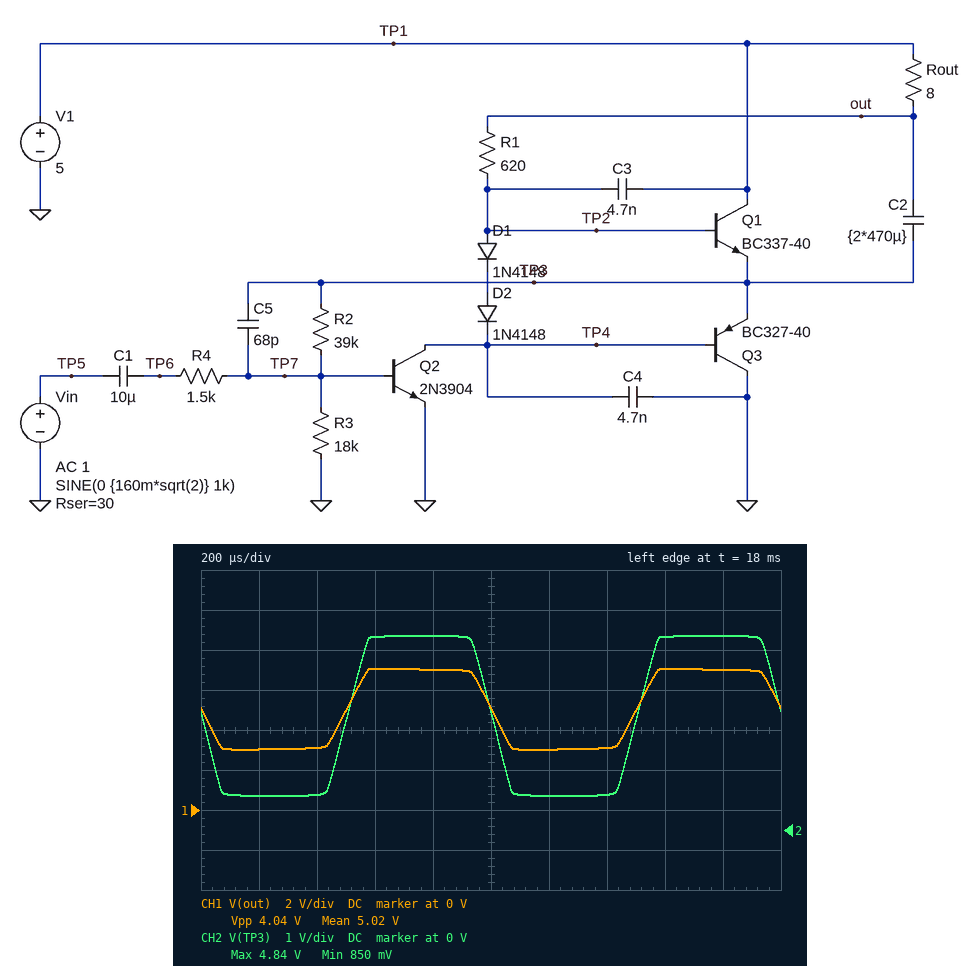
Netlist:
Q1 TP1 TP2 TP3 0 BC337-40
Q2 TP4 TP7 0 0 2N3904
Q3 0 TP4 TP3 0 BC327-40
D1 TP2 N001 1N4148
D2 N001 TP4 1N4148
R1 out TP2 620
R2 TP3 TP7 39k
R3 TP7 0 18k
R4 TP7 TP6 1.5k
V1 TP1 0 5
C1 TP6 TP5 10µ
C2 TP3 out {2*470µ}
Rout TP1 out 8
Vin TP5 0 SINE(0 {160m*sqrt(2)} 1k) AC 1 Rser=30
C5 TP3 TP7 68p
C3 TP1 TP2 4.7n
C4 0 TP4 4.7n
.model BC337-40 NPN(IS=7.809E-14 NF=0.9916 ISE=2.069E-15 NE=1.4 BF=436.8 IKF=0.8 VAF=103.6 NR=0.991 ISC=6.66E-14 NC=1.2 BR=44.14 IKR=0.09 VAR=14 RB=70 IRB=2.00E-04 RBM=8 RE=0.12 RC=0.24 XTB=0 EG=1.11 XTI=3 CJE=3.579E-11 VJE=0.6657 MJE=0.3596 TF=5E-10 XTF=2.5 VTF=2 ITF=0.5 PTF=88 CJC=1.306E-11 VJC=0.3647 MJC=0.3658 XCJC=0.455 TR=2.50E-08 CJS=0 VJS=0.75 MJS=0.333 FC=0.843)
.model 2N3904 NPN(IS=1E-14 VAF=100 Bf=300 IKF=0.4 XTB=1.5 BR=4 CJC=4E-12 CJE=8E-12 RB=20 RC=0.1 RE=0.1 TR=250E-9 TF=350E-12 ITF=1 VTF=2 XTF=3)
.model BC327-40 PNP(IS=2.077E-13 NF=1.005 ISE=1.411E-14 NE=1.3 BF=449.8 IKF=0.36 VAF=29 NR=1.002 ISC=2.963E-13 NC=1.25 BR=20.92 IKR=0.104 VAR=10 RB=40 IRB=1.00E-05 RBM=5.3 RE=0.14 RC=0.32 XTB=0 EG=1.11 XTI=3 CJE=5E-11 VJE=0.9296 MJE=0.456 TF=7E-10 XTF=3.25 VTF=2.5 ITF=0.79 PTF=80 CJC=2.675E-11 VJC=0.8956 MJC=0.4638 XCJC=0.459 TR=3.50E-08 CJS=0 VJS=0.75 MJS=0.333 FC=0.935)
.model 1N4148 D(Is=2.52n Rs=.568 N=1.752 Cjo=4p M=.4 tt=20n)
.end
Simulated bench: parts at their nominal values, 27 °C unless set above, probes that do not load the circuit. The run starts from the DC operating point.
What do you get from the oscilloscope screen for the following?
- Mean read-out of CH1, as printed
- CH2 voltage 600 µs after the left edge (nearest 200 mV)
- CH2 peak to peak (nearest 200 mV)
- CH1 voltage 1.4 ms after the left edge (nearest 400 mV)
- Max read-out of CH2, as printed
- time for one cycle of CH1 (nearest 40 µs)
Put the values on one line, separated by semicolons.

5.02 V; 4.8 V; 4.0 V; 3.2 V; 4.84 V; 1.00 ms
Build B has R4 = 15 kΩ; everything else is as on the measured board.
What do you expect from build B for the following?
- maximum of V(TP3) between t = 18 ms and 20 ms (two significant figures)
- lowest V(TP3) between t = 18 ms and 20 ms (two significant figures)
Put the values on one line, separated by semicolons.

3.1 V; 2.0 V
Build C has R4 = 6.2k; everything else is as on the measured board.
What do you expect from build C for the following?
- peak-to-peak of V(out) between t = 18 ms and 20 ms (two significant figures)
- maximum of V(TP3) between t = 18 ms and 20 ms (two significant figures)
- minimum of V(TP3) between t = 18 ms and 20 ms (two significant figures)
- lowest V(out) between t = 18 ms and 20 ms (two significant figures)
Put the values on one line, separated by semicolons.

2.5 V; 3.8 V; 1.3 V; 3.7 V
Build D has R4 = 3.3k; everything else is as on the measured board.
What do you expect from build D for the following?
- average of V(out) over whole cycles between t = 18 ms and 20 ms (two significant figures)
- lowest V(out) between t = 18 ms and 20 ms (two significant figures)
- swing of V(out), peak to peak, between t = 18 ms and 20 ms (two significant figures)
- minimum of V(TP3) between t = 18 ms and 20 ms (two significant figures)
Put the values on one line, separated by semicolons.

5.0 V; 3.2 V; 3.9 V; 880 mV
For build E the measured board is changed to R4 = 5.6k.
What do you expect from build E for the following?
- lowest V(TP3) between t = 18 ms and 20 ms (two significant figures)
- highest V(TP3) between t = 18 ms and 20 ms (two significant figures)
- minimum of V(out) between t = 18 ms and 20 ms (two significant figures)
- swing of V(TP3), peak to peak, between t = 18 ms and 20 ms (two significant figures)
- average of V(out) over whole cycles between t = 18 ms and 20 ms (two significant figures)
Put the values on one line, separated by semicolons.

1.2 V; 3.9 V; 3.6 V; 2.8 V; 5.0 V
